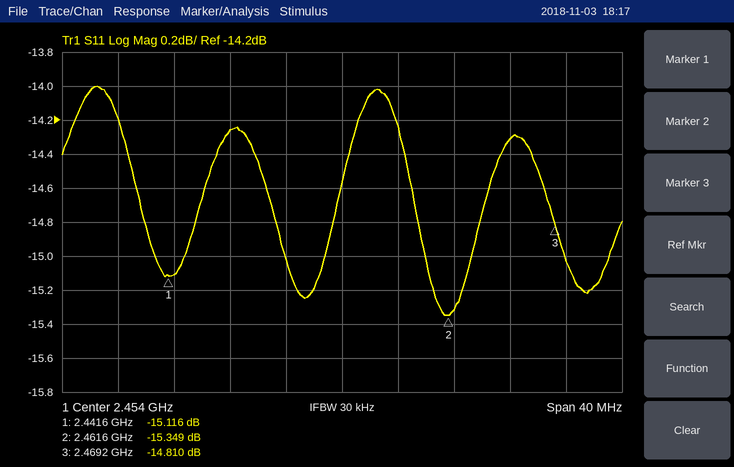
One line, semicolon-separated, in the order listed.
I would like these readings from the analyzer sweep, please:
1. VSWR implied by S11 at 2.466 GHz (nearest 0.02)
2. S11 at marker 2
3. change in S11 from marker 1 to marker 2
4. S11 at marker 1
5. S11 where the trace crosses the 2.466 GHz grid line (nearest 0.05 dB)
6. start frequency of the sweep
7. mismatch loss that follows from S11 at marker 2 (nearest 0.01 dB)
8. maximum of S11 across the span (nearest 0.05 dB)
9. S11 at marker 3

1.48; -15.349 dB; -0.233 dB; -15.116 dB; -14.30 dB; 2.434 GHz; 0.13 dB; -14.00 dB; -14.810 dB
